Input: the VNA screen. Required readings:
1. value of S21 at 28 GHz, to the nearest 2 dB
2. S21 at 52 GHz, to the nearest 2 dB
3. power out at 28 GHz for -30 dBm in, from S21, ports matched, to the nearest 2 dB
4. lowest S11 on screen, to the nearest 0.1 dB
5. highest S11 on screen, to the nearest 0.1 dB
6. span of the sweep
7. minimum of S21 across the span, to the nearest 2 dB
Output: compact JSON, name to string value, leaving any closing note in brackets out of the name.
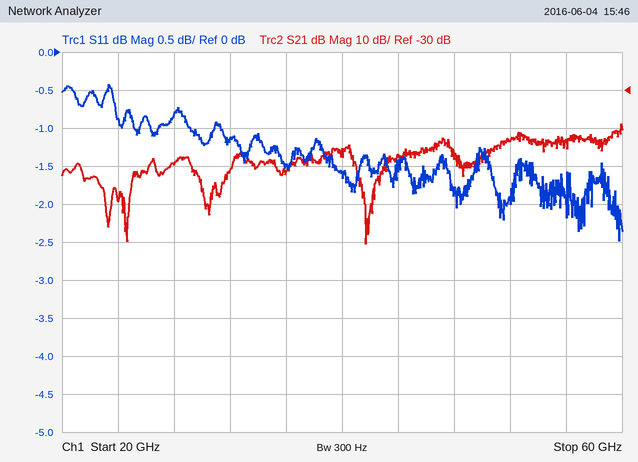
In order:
{"value of S21 at 28 GHz, to the nearest 2 dB": "-50 dB", "S21 at 52 GHz, to the nearest 2 dB": "-44 dB", "power out at 28 GHz for -30 dBm in, from S21, ports matched, to the nearest 2 dB": "-80 dBm", "lowest S11 on screen, to the nearest 0.1 dB": "-2.5 dB", "highest S11 on screen, to the nearest 0.1 dB": "-0.4 dB", "span of the sweep": "40 GHz", "minimum of S21 across the span, to the nearest 2 dB": "-70 dB"}
